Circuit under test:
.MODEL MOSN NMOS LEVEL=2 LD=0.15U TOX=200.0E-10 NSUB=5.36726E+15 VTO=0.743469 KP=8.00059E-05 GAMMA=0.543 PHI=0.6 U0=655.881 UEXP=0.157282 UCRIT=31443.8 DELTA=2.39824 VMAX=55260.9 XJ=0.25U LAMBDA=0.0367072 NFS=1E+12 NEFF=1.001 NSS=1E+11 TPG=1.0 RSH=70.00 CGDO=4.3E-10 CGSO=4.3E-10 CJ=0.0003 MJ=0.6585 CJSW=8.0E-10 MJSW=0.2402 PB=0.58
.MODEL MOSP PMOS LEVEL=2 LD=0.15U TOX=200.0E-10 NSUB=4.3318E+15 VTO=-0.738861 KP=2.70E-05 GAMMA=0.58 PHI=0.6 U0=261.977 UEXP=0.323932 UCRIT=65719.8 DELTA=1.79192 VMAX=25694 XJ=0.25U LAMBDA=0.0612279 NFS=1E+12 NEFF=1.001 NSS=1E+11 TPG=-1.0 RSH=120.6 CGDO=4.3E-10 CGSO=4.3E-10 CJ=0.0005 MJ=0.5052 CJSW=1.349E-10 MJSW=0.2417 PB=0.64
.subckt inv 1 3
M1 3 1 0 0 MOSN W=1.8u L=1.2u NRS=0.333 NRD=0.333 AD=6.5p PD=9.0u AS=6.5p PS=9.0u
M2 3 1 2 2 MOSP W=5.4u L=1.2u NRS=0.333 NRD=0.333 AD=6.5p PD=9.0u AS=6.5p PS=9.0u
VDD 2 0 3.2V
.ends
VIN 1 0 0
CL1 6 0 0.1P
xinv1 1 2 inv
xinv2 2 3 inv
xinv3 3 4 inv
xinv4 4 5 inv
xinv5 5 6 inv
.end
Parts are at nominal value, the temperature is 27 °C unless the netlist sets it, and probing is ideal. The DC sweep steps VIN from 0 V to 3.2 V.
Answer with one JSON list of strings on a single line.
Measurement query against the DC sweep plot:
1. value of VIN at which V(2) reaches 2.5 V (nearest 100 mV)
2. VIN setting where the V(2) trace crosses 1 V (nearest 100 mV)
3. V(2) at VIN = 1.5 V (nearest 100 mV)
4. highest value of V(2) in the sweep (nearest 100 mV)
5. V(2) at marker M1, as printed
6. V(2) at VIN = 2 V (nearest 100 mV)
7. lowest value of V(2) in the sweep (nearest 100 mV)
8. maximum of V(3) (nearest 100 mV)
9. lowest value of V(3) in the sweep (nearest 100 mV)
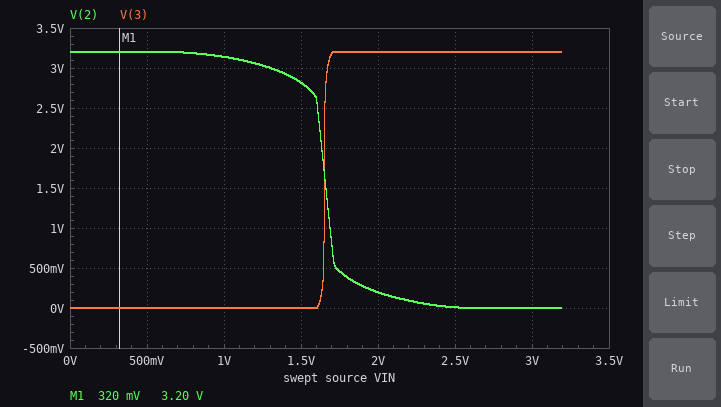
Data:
["1.6 V", "1.7 V", "2.8 V", "3.2 V", "3.20 V", "200 mV", "0 V", "3.2 V", "0 V"]
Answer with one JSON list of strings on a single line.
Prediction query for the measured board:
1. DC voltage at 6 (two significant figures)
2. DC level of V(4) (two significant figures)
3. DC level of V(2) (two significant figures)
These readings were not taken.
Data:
["3.2 V", "3.2 V", "3.2 V"]
